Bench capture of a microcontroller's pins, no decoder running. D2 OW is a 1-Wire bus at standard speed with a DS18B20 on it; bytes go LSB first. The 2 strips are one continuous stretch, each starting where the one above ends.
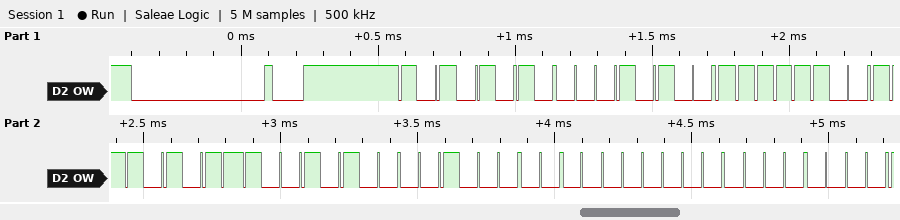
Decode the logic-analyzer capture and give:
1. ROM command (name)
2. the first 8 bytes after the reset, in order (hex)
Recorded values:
Match ROM
55 28 3F D7 29 04 00 00
